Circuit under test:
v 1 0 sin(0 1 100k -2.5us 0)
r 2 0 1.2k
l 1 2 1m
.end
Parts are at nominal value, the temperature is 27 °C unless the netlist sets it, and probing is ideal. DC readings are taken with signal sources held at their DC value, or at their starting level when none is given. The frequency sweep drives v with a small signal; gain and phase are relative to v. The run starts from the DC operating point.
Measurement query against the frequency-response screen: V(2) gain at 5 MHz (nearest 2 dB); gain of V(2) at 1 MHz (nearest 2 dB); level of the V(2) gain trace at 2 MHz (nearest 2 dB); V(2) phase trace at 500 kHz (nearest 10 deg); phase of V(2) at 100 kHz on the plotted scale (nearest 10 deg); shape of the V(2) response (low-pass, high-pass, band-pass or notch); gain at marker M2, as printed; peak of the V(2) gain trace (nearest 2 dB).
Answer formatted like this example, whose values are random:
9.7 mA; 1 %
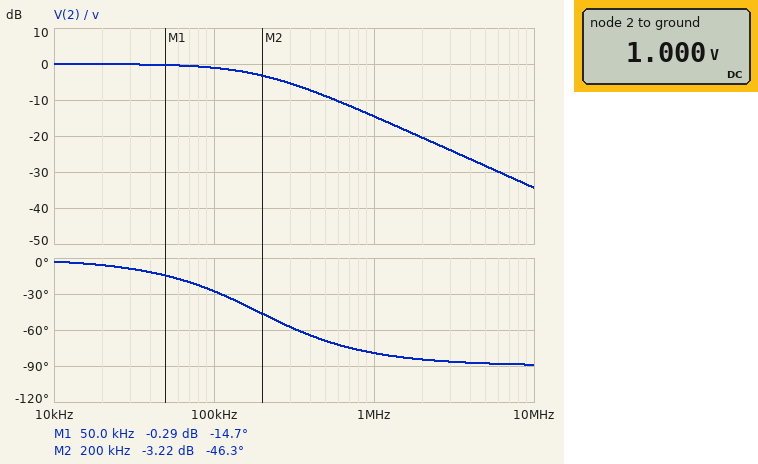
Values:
-28 dB; -14 dB; -20 dB; -70 deg; -30 deg; low-pass; -3.22 dB; 0 dB
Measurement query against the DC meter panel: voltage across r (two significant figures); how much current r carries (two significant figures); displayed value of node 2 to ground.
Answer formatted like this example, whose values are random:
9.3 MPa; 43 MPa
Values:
1.0 V; 830 µA; 1.000 V
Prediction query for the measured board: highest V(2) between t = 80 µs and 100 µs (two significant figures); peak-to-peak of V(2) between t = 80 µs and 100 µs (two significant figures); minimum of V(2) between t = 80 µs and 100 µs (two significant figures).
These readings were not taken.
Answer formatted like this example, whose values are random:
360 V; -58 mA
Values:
890 mV; 1.8 V; -890 mV
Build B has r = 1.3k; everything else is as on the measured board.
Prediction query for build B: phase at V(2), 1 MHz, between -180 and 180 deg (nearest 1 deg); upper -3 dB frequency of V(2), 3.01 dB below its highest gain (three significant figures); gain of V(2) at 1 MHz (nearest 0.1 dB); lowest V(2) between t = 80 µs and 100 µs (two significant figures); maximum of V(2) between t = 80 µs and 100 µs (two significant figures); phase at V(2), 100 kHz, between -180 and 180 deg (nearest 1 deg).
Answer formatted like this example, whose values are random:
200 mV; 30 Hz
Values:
-78 deg; 207 kHz; -13.9 dB; -900 mV; 900 mV; -26 deg
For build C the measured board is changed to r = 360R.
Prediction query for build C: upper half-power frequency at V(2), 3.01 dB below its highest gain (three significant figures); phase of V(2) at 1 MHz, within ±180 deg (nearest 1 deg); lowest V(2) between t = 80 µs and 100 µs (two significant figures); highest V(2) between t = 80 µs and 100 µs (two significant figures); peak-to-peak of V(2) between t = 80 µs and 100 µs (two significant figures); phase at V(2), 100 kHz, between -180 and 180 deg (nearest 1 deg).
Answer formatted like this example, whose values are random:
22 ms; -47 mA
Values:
57.3 kHz; -87 deg; -500 mV; 500 mV; 990 mV; -60 deg
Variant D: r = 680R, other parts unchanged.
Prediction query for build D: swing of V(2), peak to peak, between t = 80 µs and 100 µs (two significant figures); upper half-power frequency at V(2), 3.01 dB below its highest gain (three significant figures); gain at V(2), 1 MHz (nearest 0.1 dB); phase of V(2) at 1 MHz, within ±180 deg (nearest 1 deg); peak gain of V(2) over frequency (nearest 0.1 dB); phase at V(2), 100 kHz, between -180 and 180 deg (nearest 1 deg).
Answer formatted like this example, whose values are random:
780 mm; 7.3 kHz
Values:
1.5 V; 108 kHz; -19.4 dB; -84 deg; 0 dB; -43 deg
